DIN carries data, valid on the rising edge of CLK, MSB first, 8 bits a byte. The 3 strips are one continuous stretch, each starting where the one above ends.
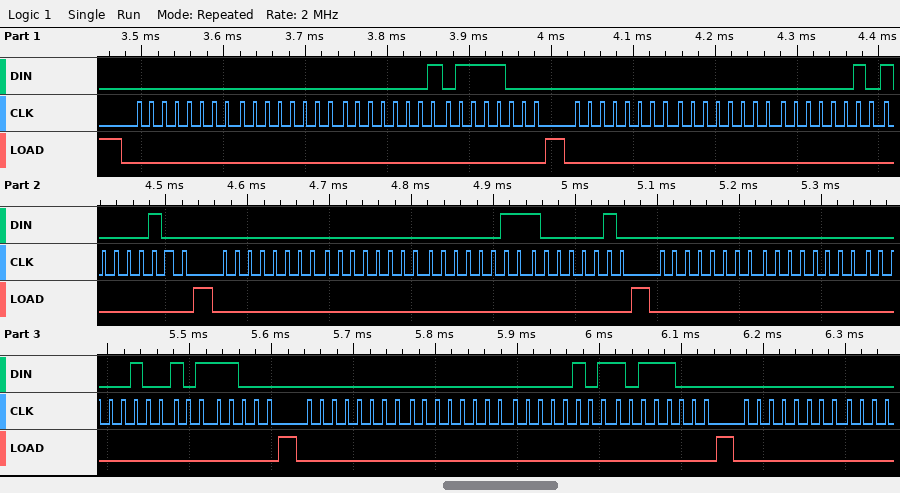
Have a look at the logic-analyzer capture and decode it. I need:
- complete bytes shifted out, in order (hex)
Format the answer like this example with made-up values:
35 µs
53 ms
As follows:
00 00 01 78 00 00 02 84 00 00 03 82 00 00 04 B8 00 00 05 B8 00
